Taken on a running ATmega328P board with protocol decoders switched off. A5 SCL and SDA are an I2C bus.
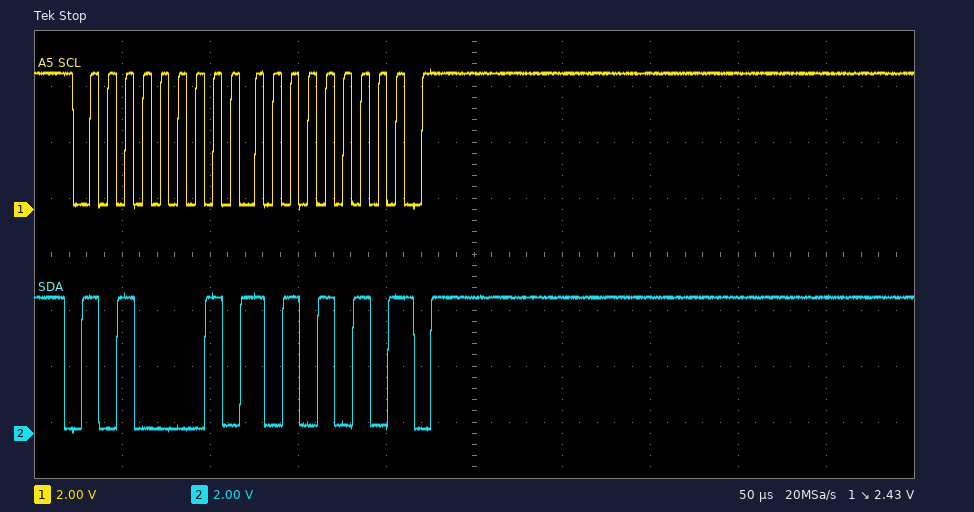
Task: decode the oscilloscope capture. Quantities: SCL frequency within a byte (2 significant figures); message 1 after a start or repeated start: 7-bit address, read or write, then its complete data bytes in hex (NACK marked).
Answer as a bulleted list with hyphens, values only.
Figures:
- 100 kHz
- 0x50 read: AA NACK
